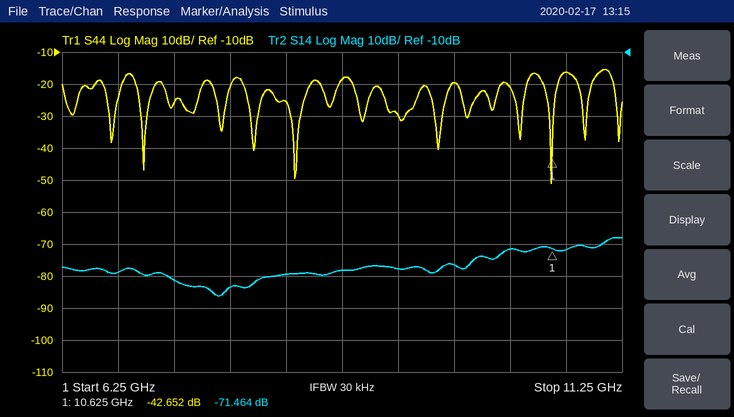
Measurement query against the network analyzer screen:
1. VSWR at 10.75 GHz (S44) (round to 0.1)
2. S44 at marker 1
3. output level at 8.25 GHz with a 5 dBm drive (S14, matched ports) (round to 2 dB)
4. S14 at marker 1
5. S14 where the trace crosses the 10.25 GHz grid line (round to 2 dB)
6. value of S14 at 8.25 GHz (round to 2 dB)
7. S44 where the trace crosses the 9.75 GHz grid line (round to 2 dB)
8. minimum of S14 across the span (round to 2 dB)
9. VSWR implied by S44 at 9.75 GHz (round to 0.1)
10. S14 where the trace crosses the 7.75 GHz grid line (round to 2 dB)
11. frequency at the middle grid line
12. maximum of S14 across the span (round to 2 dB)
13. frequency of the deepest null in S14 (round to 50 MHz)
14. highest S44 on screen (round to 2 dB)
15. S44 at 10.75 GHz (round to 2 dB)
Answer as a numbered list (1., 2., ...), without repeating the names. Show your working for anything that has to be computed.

1. |Γ| = 10^(-16/20) = 0.1585; VSWR = (1 + 0.1585)/(1 − 0.1585) ≈ 1.4
2. -42.652 dB
3. 5 dBm + (-80 dB) = -74 dBm
4. -71.464 dB
5. -72 dB
6. -80 dB
7. -20 dB
8. -86 dB
9. |Γ| = 10^(-20/20) = 0.1000; VSWR = (1 + 0.1000)/(1 − 0.1000) ≈ 1.2
10. -84 dB
11. 8.75 GHz
12. -68 dB
13. 7.65 GHz
14. -16 dB
15. -16 dB
